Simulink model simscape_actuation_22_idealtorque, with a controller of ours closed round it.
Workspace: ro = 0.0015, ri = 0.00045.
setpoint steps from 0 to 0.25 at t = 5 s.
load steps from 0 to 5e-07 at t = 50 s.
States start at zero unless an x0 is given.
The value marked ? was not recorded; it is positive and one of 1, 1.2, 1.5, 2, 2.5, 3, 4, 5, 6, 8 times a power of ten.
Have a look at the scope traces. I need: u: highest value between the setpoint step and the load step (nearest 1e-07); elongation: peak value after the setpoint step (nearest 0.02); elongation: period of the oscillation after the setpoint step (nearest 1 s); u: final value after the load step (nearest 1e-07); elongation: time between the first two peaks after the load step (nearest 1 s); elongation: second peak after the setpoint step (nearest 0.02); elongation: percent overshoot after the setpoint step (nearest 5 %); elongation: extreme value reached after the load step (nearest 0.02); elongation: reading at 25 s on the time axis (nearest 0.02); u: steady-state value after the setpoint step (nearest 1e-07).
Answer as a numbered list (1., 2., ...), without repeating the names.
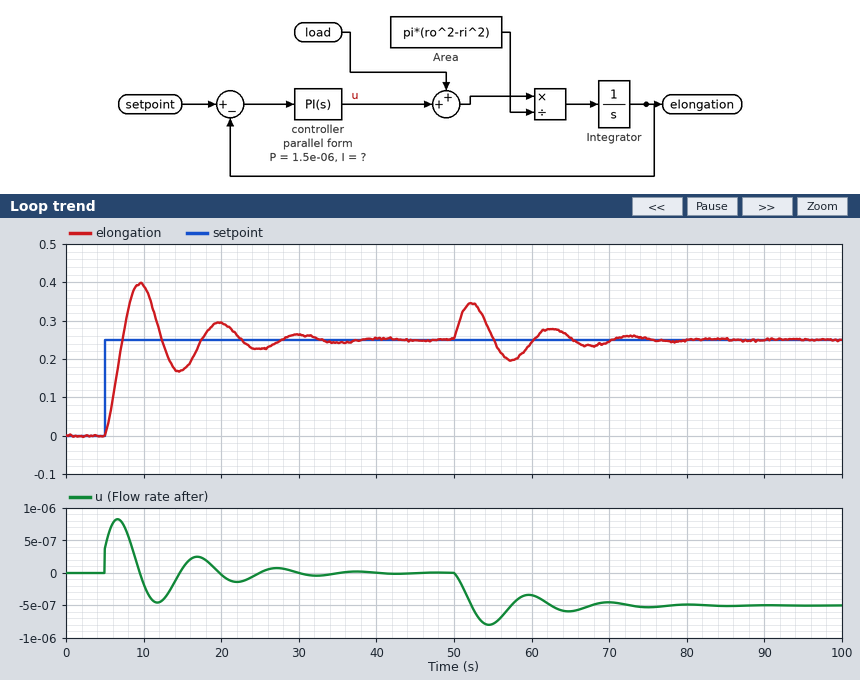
1. 0.0000008
2. 0.40
3. 10 s
4. -0.0000005
5. 10 s
6. 0.30
7. 60 %
8. 0.34
9. 0.22
10. 0.0000000
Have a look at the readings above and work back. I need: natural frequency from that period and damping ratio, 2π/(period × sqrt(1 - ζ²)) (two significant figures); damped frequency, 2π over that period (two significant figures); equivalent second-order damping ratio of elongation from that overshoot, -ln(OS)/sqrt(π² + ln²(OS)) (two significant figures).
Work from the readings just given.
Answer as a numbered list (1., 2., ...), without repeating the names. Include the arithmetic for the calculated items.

1. 2π / (10 × sqrt(1 - 0.16²)) = 0.64 rad/s
2. 2π / 10 = 0.63 rad/s
3. ln(0.6) = -0.511; 0.511 / sqrt(9.870 + 0.261) = 0.16
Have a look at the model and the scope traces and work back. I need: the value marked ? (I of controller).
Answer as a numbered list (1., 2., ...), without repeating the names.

1. 2.5e-06
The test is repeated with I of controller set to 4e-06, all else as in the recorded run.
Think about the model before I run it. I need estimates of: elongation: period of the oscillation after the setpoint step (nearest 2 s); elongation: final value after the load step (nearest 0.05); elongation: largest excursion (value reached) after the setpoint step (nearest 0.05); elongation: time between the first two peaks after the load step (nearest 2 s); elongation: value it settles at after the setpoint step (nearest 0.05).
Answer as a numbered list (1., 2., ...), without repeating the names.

1. 8 s
2. 0.25
3. 0.40
4. 8 s
5. 0.25
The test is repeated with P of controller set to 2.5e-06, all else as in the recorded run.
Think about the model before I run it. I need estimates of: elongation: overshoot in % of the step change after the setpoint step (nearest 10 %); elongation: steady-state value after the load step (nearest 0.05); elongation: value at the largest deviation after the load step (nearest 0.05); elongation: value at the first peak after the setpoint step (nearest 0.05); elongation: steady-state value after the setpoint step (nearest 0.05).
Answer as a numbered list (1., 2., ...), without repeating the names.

1. 40 %
2. 0.25
3. 0.35
4. 0.35
5. 0.25
